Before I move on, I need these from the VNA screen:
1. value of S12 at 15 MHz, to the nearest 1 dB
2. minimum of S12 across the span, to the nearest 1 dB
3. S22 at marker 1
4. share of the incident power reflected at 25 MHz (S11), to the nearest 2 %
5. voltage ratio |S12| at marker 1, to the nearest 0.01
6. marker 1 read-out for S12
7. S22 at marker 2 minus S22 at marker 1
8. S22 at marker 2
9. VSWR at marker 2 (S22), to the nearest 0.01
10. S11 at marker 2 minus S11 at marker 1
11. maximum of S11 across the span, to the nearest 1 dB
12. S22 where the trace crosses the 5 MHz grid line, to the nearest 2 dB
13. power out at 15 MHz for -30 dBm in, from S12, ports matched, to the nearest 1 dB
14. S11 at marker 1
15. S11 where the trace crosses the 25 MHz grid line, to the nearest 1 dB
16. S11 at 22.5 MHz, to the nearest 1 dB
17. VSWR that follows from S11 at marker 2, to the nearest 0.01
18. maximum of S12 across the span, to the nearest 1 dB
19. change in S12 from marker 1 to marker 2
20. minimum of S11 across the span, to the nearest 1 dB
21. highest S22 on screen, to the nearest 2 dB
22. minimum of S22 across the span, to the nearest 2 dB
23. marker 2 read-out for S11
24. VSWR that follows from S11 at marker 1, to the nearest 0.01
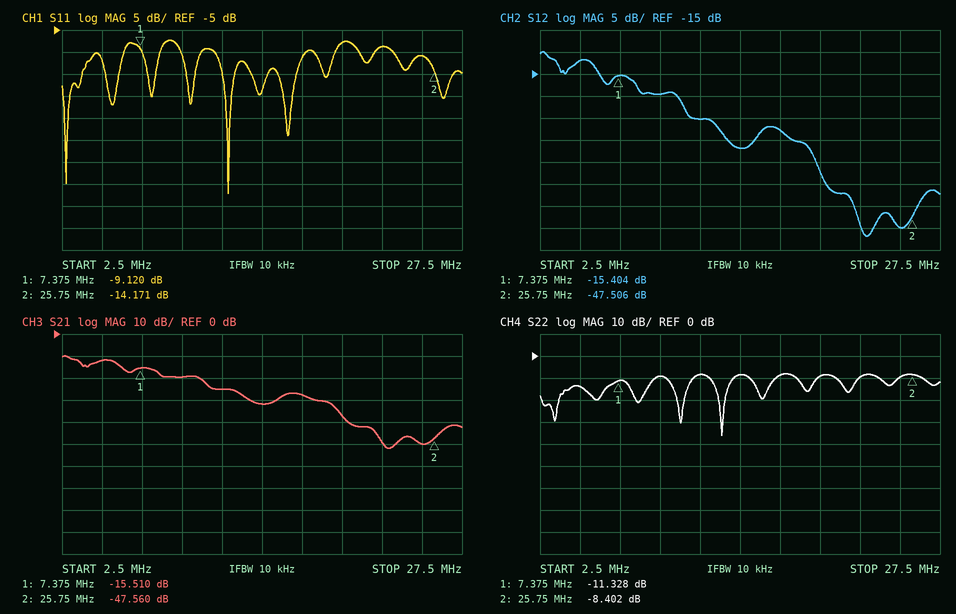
-32 dB
-52 dB
-11.328 dB
8 %
0.17
-15.404 dB
2.926 dB
-8.402 dB
2.23
-5.051 dB
-7 dB
-14 dB
-62 dBm
-9.120 dB
-11 dB
-9 dB
1.49
-10 dB
-32.102 dB
-42 dB
-8 dB
-36 dB
-14.171 dB
2.08
